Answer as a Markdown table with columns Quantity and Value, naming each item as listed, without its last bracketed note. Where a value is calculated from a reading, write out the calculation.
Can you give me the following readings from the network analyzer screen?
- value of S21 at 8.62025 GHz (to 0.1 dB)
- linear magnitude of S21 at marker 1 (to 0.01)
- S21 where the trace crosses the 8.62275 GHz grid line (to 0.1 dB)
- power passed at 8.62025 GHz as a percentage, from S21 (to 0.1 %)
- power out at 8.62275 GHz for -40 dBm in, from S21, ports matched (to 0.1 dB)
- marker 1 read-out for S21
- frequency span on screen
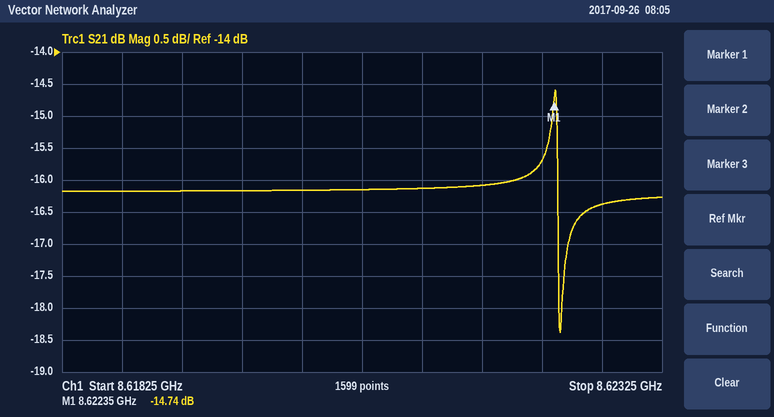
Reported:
| Quantity | Value |
|---|---|
| value of S21 at 8.62025 GHz | -16.2 dB |
| linear magnitude of S21 at marker 1 | 10^(-14.74/20) ≈ 0.18 |
| S21 where the trace crosses the 8.62275 GHz grid line | -16.4 dB |
| power passed at 8.62025 GHz as a percentage, from S21 | 10^(-16.2/10) ≈ 2.4 % |
| power out at 8.62275 GHz for -40 dBm in, from S21, ports matched | -40 dBm + (-16.4 dB) = -56.4 dBm |
| marker 1 read-out for S21 | -14.74 dB |
| frequency span on screen | 5 MHz |
